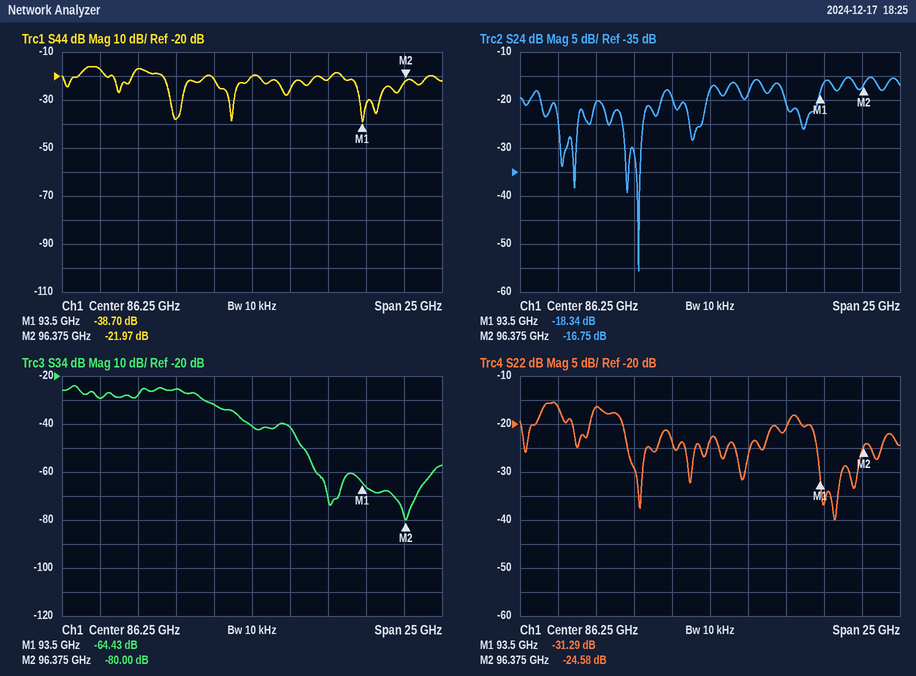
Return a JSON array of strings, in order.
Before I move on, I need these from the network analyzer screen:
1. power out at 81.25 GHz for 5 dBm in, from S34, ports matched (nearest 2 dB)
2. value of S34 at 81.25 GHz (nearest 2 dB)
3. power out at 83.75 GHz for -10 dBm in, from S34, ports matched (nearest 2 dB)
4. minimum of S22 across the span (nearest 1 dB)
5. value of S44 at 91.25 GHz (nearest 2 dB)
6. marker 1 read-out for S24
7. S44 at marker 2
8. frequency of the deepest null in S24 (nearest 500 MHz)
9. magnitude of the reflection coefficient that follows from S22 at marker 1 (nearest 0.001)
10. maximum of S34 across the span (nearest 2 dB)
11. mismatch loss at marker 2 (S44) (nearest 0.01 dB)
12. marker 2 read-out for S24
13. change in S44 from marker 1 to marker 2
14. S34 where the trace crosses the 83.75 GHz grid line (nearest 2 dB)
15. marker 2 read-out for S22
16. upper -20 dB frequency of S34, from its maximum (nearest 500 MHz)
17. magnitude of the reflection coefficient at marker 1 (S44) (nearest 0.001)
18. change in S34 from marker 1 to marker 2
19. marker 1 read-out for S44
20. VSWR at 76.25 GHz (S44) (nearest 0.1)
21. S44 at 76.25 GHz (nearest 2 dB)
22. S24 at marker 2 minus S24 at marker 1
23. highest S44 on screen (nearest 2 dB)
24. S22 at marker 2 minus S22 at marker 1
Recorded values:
["-20 dBm", "-26 dB", "-42 dBm", "-40 dB", "-22 dB", "-18.34 dB", "-21.97 dB", "81.5 GHz", "0.027", "-24 dB", "0.03 dB", "-16.75 dB", "16.73 dB", "-32 dB", "-24.58 dB", "89.0 GHz", "0.012", "-15.57 dB", "-38.70 dB", "1.3", "-18 dB", "1.59 dB", "-16 dB", "6.71 dB"]
